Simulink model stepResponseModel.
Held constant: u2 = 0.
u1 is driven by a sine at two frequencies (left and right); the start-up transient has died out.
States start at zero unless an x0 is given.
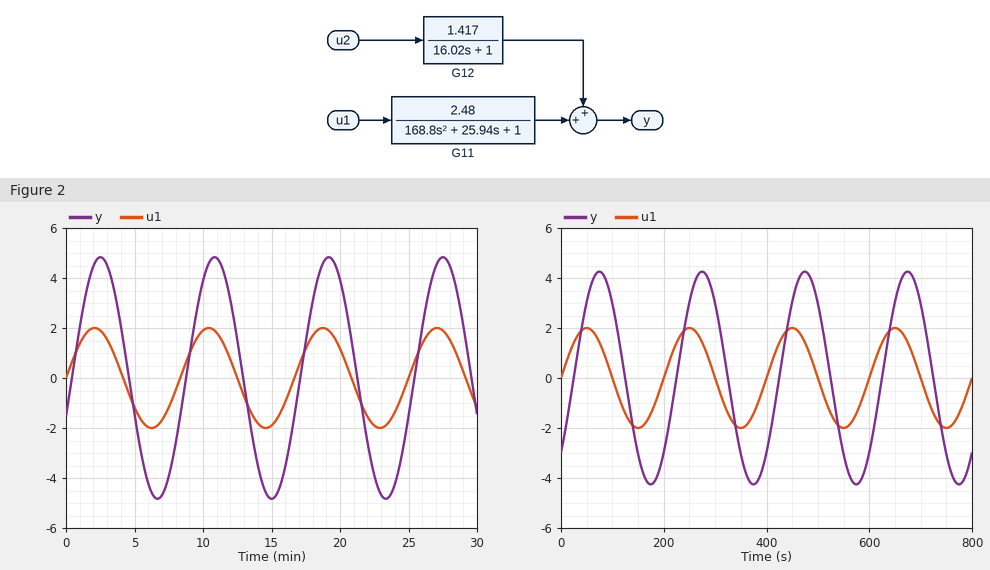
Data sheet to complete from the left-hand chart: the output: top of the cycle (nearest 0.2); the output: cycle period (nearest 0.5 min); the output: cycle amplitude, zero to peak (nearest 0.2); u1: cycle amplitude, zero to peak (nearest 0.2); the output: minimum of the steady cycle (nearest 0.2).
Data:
4.8
8.5 min
4.8
2.0
-4.8
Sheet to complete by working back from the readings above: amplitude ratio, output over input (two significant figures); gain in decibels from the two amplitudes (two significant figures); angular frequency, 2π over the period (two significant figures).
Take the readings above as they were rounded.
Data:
2.4
7.6 dB
0.74 rad/min
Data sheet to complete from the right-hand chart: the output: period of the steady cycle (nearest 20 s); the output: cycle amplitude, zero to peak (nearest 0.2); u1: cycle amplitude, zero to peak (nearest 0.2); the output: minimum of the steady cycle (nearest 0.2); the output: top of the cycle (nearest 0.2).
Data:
200 s
4.2
2.0
-4.2
4.2
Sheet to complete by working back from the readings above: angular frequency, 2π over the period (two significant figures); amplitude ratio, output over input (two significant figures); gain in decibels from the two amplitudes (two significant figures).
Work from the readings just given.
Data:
0.031 rad/s
2.1
6.4 dB
